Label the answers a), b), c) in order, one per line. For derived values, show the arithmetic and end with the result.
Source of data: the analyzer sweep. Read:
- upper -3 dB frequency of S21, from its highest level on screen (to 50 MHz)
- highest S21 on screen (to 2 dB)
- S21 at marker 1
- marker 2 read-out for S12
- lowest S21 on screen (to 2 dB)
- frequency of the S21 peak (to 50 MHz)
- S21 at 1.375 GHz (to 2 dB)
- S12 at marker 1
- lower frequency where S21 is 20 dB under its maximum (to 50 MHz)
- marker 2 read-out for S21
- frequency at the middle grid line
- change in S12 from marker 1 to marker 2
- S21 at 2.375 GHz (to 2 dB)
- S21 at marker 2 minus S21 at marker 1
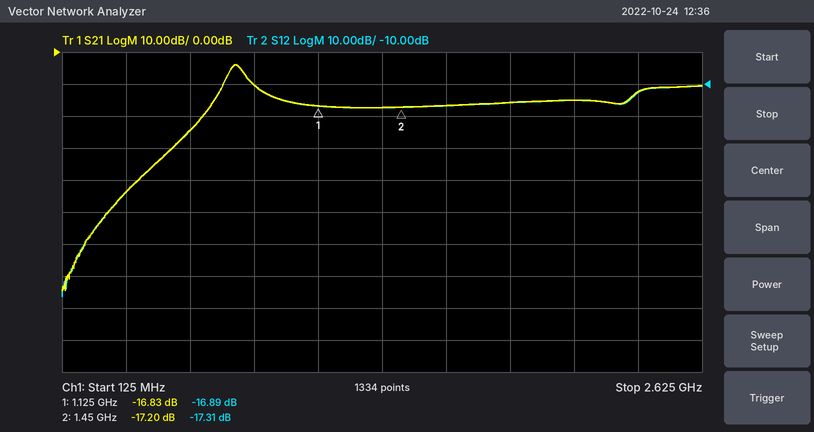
a) 850 MHz
b) -4 dB
c) -16.83 dB
d) -17.31 dB
e) -74 dB
f) 800 MHz
g) -18 dB
h) -16.89 dB
i) 650 MHz
j) -17.20 dB
k) 1.375 GHz
l) -17.31 − (-16.89) = -0.42 dB
m) -12 dB
n) -17.2 − (-16.83) = -0.37 dB
